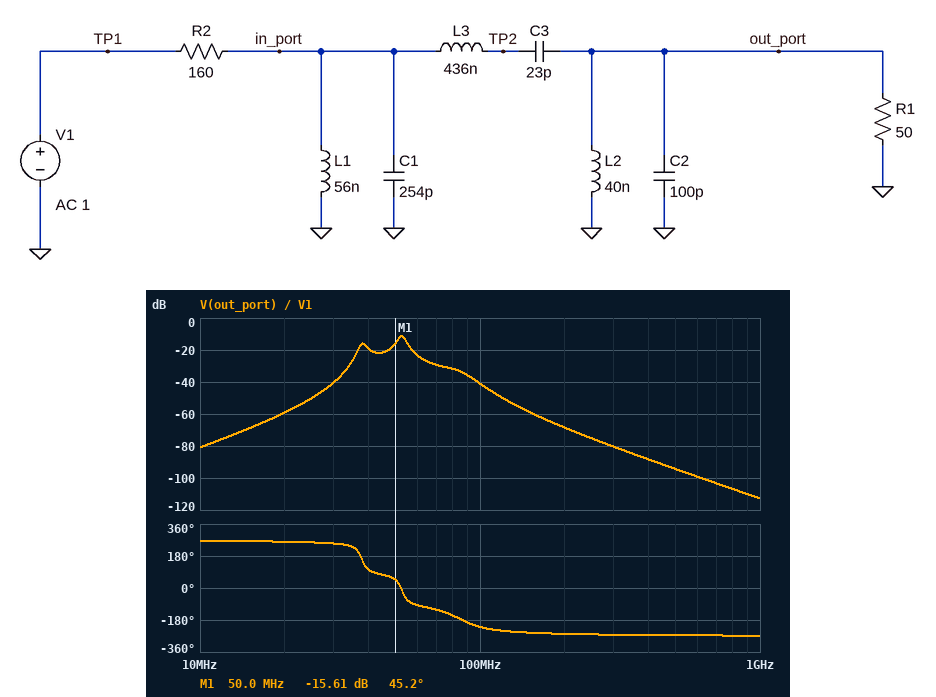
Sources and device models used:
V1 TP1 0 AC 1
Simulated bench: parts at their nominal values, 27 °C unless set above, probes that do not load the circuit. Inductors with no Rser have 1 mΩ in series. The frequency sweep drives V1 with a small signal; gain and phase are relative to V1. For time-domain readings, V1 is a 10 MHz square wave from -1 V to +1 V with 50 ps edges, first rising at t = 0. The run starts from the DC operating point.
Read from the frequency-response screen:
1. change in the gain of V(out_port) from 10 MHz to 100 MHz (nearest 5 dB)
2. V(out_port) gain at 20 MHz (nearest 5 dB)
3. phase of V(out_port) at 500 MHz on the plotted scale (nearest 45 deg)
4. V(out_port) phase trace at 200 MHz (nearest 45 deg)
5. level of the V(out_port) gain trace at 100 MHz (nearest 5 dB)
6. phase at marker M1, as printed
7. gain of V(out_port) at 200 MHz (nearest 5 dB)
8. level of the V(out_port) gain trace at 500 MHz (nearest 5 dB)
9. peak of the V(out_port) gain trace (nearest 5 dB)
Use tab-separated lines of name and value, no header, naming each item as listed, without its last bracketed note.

change in the gain of V(out_port) from 10 MHz to 100 MHz	40 dB
V(out_port) gain at 20 MHz	-60 dB
phase of V(out_port) at 500 MHz on the plotted scale	-270 deg
V(out_port) phase trace at 200 MHz	-270 deg
level of the V(out_port) gain trace at 100 MHz	-40 dB
phase at marker M1, as printed	45.2 deg
gain of V(out_port) at 200 MHz	-70 dB
level of the V(out_port) gain trace at 500 MHz	-95 dB
peak of the V(out_port) gain trace	-10 dB
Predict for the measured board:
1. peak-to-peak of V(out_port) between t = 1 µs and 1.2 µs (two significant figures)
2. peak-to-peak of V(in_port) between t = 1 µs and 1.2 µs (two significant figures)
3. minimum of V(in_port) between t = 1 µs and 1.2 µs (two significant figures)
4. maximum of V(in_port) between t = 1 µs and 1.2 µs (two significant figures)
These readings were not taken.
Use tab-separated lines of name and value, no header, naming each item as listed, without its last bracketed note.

peak-to-peak of V(out_port) between t = 1 µs and 1.2 µs	100 mV
peak-to-peak of V(in_port) between t = 1 µs and 1.2 µs	280 mV
minimum of V(in_port) between t = 1 µs and 1.2 µs	-140 mV
maximum of V(in_port) between t = 1 µs and 1.2 µs	140 mV
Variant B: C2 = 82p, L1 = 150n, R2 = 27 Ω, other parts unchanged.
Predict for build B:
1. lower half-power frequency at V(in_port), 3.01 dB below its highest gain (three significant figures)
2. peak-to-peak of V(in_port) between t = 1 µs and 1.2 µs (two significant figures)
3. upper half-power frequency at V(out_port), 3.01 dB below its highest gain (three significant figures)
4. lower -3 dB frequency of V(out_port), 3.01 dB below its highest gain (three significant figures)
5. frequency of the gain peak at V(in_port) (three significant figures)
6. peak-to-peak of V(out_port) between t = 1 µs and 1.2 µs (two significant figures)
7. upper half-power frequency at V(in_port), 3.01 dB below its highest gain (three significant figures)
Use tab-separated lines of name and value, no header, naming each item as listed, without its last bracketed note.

lower half-power frequency at V(in_port), 3.01 dB below its highest gain	16.2 MHz
peak-to-peak of V(in_port) between t = 1 µs and 1.2 µs	1.9 V
upper half-power frequency at V(out_port), 3.01 dB below its highest gain	51.9 MHz
lower -3 dB frequency of V(out_port), 3.01 dB below its highest gain	47.5 MHz
frequency of the gain peak at V(in_port)	24.3 MHz
peak-to-peak of V(out_port) between t = 1 µs and 1.2 µs	430 mV
upper half-power frequency at V(in_port), 3.01 dB below its highest gain	35.1 MHz
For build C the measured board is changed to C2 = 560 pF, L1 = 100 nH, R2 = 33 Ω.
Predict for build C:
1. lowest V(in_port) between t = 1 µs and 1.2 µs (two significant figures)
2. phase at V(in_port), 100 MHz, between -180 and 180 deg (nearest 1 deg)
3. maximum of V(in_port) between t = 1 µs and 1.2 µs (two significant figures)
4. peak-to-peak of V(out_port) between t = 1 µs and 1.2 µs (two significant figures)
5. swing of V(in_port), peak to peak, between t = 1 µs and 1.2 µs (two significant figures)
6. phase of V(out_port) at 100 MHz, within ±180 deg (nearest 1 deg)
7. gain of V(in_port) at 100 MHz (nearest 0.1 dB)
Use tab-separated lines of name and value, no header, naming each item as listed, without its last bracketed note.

lowest V(in_port) between t = 1 µs and 1.2 µs	-740 mV
phase at V(in_port), 100 MHz, between -180 and 180 deg	-78 deg
maximum of V(in_port) between t = 1 µs and 1.2 µs	740 mV
peak-to-peak of V(out_port) between t = 1 µs and 1.2 µs	290 mV
swing of V(in_port), peak to peak, between t = 1 µs and 1.2 µs	1.5 V
phase of V(out_port) at 100 MHz, within ±180 deg	106 deg
gain of V(in_port) at 100 MHz	-13.4 dB
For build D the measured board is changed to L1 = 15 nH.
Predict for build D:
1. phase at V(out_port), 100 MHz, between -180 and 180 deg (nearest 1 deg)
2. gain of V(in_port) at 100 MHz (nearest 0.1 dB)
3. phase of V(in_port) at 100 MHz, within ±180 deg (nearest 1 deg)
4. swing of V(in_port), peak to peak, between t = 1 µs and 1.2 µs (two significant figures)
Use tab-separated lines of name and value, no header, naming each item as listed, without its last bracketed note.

phase at V(out_port), 100 MHz, between -180 and 180 deg	146 deg
gain of V(in_port) at 100 MHz	-17.8 dB
phase of V(in_port) at 100 MHz, within ±180 deg	-82 deg
swing of V(in_port), peak to peak, between t = 1 µs and 1.2 µs	140 mV
